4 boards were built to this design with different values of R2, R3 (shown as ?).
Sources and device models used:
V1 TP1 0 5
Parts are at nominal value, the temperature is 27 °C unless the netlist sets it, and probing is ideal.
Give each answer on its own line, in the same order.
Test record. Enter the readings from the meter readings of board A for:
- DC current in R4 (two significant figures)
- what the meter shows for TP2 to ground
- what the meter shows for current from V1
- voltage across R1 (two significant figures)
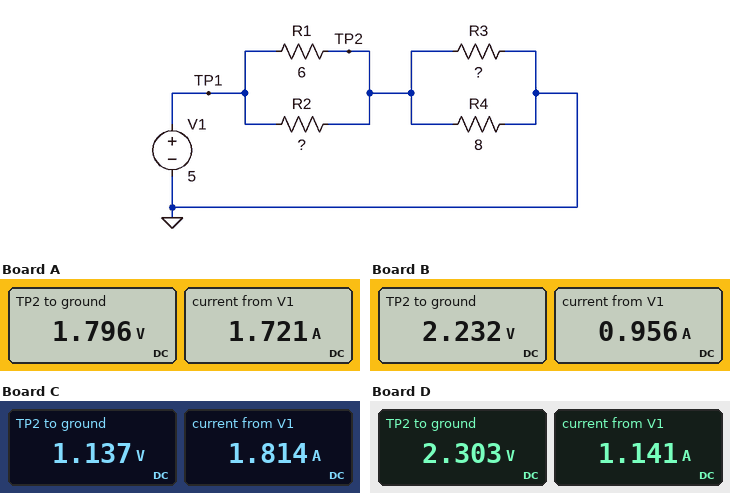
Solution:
220 mA
1.796 V
1.721 A
3.2 V
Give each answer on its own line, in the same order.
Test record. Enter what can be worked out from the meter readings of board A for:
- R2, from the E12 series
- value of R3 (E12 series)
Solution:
2.7 Ω
1.2 Ω
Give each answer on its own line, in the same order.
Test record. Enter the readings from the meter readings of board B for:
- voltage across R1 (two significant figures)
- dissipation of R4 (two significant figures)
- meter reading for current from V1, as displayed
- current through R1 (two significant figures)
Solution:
2.8 V
620 mW
0.956 A
460 mA
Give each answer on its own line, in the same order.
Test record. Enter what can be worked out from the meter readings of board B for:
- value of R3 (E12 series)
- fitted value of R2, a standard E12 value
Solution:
3.3 Ω
5.6 Ω
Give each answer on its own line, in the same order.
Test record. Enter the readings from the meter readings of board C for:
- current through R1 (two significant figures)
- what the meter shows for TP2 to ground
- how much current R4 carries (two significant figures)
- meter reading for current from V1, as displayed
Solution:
640 mA
1.137 V
140 mA
1.814 A
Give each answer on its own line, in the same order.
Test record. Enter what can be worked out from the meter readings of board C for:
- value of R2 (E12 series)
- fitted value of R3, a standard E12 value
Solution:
3.3 Ω
0.68 Ω
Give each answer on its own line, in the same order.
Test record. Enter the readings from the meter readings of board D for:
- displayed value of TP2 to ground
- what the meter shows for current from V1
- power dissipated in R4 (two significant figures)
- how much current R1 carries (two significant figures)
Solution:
2.303 V
1.141 A
660 mW
450 mA
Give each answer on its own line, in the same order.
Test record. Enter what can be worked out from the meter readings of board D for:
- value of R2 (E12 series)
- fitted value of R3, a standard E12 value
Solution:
3.9 Ω
2.7 Ω
